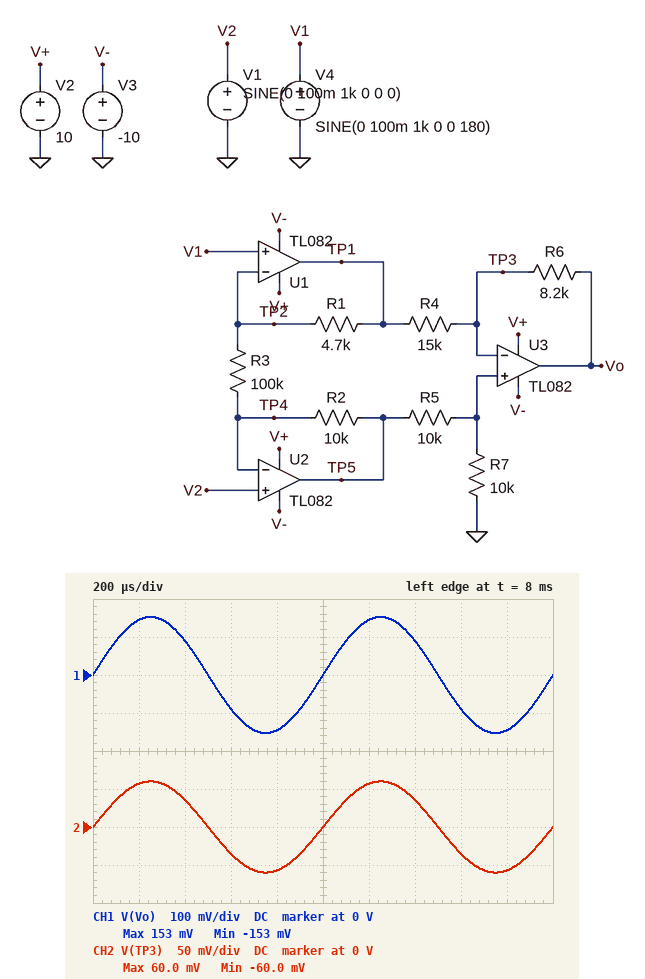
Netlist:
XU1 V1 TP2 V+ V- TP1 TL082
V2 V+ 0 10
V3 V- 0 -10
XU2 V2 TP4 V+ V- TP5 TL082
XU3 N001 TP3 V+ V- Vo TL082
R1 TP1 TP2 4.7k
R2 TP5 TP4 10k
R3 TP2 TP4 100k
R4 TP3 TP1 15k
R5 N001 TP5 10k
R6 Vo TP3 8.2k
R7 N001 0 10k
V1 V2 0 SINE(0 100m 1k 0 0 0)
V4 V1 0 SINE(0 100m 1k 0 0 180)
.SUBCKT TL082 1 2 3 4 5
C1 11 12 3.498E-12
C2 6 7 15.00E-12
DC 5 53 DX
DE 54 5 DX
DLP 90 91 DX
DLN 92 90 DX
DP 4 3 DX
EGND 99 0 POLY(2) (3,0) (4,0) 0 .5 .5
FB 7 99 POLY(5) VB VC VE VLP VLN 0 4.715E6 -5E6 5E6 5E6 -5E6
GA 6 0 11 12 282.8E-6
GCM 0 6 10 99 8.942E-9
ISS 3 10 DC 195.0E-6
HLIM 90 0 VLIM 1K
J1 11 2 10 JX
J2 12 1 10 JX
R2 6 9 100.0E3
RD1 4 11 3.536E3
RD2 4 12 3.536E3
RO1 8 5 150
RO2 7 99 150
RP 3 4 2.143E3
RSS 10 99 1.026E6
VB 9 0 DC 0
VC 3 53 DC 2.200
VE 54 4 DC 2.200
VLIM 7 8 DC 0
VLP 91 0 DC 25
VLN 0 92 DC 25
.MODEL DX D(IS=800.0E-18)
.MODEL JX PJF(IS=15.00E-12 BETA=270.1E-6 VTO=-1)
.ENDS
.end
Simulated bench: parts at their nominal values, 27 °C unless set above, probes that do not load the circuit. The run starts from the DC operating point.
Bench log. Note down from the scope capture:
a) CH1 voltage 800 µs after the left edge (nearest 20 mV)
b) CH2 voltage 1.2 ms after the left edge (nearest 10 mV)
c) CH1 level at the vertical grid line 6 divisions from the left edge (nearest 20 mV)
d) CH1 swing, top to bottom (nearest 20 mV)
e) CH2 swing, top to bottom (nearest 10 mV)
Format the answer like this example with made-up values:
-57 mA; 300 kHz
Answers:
-140 mV; 60 mV; 140 mV; 300 mV; 120 mV
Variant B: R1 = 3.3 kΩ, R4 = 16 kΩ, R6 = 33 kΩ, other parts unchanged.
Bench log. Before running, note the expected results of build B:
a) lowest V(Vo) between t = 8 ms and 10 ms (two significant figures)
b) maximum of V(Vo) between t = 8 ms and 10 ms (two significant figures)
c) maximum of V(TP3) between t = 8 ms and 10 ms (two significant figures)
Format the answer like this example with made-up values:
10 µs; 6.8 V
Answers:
-400 mV; 400 mV; 60 mV
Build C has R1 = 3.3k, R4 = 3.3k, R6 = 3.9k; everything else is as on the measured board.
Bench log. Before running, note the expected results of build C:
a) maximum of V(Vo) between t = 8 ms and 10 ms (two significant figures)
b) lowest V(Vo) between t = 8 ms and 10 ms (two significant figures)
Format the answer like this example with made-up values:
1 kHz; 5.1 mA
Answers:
260 mV; -260 mV
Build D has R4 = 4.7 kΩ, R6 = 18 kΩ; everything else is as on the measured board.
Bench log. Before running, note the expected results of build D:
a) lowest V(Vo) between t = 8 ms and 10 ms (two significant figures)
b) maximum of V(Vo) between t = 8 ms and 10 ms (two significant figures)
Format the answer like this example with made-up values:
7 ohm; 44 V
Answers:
-710 mV; 710 mV
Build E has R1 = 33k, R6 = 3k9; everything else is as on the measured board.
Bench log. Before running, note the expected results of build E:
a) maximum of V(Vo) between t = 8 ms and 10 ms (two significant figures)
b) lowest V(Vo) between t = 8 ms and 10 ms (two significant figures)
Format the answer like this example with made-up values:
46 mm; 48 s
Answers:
120 mV; -120 mV
